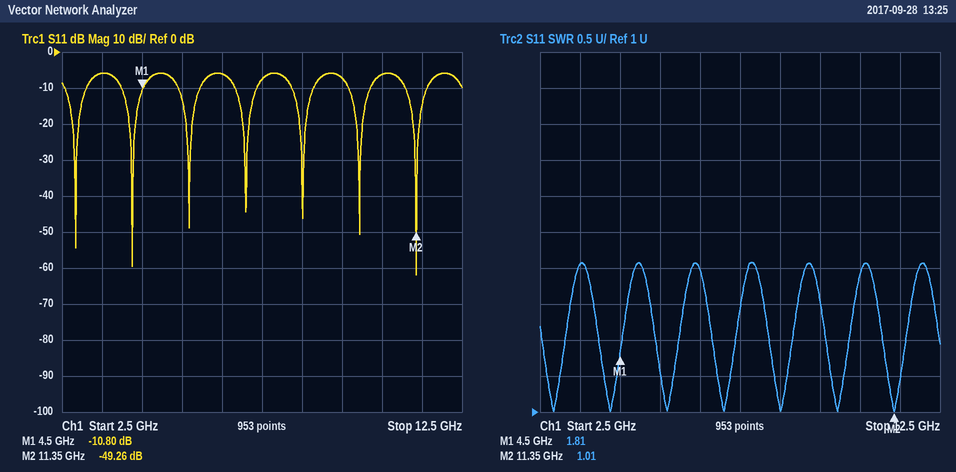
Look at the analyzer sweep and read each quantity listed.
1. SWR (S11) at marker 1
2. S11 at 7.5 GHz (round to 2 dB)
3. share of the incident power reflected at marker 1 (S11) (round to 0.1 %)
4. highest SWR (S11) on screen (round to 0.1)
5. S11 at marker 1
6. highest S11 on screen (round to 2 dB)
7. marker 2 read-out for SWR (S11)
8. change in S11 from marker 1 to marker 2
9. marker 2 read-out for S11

1.81
-8 dB
8.3 %
3.1
-10.80 dB
-6 dB
1.01
-38.46 dB
-49.26 dB
